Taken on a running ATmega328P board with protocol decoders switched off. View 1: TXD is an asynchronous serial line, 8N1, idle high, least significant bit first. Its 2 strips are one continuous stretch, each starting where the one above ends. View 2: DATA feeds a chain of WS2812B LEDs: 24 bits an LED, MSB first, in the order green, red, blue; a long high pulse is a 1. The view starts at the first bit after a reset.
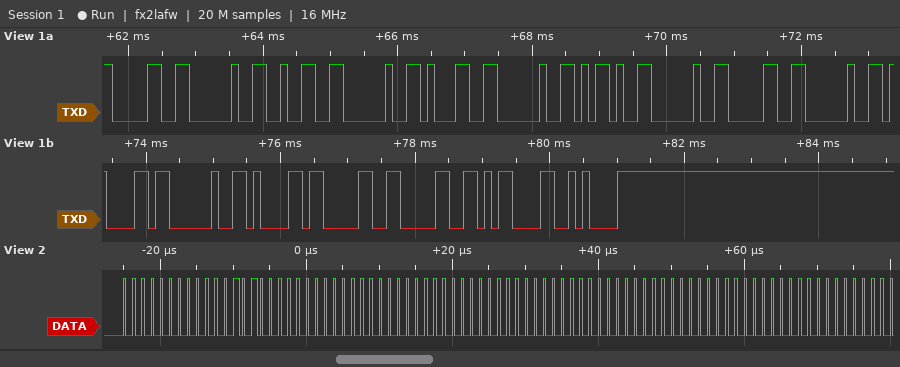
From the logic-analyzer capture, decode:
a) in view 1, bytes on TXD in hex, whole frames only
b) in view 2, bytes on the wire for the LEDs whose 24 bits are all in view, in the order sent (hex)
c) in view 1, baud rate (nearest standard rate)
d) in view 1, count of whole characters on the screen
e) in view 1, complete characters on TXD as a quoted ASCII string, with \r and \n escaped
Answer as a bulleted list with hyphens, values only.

- 0x30 0x20 0x32 0x20 0x31 0x20 0x2D 0x20 0x30 0x20 0x61 0x20 0x61 0x30 0x30 0x0D 0x0A
- 00 0A 00 00 00 00 00 00 00
- 9600 baud
- 17
- "0 2 1 - 0 a a00\r\n"
